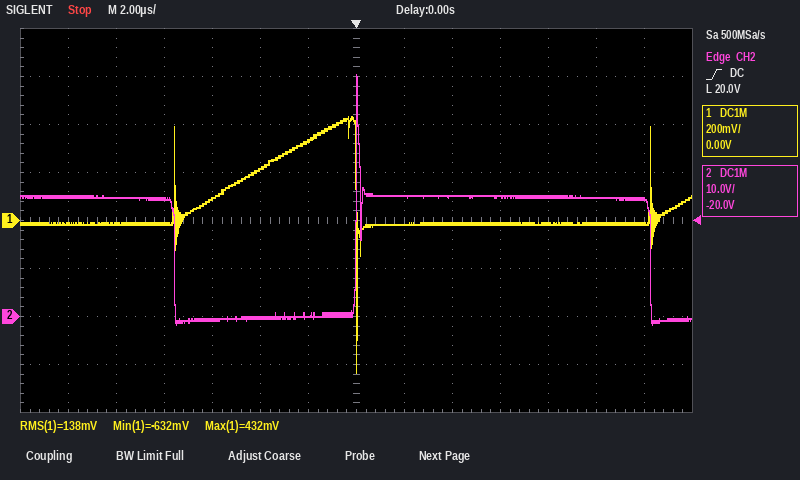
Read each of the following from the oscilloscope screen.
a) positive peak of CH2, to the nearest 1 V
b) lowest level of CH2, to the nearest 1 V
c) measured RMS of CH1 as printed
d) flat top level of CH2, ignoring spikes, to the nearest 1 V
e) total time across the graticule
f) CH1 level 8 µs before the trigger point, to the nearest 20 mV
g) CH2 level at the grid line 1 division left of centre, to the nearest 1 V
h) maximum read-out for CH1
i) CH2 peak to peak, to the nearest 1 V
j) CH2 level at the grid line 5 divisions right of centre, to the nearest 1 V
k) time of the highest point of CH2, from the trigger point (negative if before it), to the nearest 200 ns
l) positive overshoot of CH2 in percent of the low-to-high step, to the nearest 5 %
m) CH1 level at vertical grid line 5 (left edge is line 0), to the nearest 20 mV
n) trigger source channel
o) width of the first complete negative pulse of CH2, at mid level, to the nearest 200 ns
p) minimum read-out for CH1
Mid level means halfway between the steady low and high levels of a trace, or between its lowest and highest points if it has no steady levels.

50 V
-2 V
138 mV
25 V
28 µs
-20 mV
0 V
432 mV
52 V
25 V
0.0 µs
100 %
220 mV
CH2
7.6 µs
-632 mV
